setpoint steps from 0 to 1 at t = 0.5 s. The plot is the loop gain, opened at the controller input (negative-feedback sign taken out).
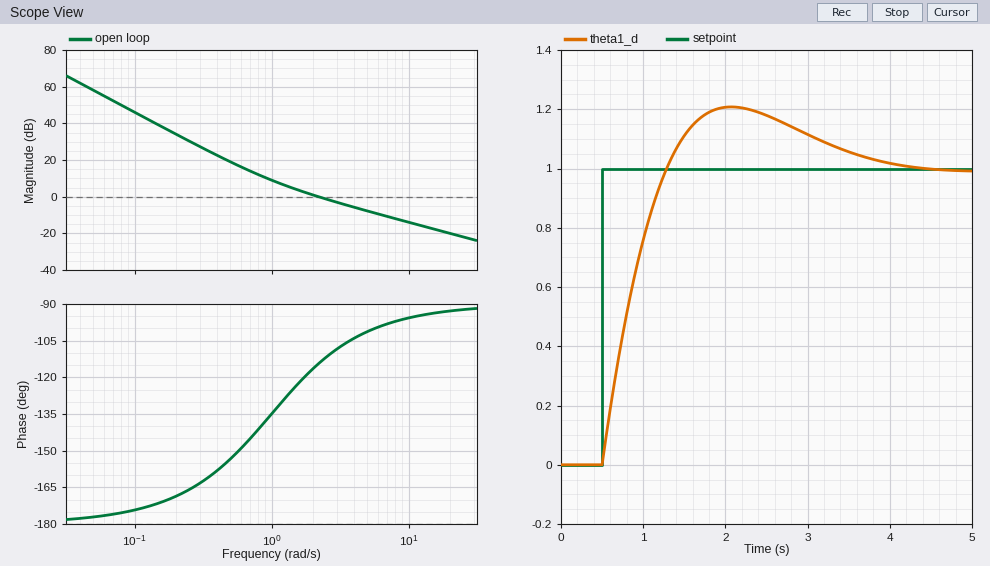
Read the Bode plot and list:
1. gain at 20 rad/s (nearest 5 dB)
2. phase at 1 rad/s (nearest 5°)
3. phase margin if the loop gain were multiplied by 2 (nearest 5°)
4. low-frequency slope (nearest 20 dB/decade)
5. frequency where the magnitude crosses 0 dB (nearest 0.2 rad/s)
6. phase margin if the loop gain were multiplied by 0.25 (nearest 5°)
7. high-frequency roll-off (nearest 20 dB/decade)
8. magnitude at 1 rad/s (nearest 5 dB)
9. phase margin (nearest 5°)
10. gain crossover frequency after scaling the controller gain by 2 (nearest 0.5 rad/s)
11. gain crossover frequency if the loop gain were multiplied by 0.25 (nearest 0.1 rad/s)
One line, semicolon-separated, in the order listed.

-20 dB; -135°; 75°; -40 dB/decade; 2.2 rad/s; 40°; -20 dB/decade; 10 dB; 65°; 4.0 rad/s; 0.8 rad/s
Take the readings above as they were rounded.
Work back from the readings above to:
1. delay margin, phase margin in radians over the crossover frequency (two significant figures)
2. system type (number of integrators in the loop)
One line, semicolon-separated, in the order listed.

0.52 s; 2
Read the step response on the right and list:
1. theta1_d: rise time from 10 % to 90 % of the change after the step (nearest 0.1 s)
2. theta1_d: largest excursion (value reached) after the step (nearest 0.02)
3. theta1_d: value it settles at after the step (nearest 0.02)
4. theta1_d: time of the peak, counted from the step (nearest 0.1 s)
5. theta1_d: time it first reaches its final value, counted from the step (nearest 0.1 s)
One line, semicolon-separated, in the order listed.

0.6 s; 1.20; 1.00; 1.6 s; 0.8 s
